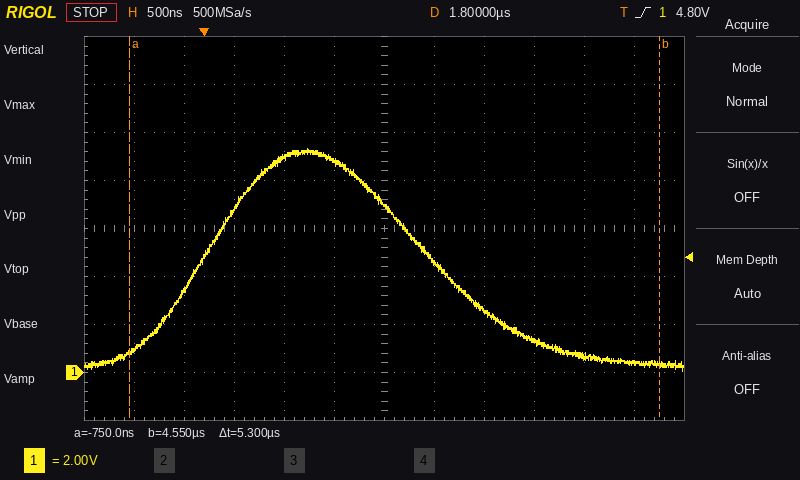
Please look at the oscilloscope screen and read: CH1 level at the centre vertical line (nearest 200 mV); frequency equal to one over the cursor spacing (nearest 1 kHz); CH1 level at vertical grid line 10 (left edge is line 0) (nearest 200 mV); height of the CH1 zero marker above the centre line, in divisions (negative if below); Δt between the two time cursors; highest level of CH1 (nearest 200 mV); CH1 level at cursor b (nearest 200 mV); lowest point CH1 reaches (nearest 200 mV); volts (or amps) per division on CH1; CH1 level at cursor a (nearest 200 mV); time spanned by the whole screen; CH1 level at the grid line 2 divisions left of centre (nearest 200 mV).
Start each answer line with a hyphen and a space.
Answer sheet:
- 7.0 V
- 189 kHz
- 600 mV
- -3.0 div
- 5.3 µs
- 9.4 V
- 400 mV
- 0.0 V
- 2 V
- 800 mV
- 6 µs
- 9.0 V
